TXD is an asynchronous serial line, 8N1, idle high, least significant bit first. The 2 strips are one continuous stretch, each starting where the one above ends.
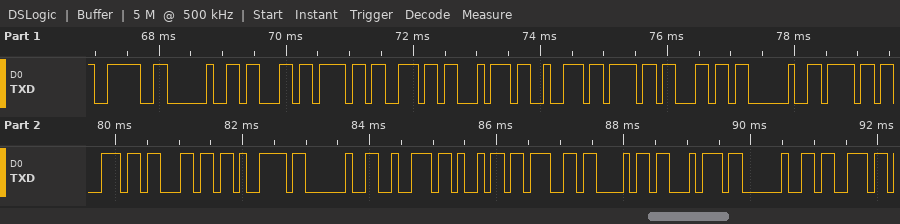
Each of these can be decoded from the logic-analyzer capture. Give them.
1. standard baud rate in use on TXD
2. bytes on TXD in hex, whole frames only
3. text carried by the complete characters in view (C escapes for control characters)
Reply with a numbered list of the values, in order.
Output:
1. 9600 baud
2. 3E 20 63 6F 6E 74 72 6F 6C 20 6F 6E 6C 79 20 72 69 67 68 74 20 73
3. "> control only right s"
